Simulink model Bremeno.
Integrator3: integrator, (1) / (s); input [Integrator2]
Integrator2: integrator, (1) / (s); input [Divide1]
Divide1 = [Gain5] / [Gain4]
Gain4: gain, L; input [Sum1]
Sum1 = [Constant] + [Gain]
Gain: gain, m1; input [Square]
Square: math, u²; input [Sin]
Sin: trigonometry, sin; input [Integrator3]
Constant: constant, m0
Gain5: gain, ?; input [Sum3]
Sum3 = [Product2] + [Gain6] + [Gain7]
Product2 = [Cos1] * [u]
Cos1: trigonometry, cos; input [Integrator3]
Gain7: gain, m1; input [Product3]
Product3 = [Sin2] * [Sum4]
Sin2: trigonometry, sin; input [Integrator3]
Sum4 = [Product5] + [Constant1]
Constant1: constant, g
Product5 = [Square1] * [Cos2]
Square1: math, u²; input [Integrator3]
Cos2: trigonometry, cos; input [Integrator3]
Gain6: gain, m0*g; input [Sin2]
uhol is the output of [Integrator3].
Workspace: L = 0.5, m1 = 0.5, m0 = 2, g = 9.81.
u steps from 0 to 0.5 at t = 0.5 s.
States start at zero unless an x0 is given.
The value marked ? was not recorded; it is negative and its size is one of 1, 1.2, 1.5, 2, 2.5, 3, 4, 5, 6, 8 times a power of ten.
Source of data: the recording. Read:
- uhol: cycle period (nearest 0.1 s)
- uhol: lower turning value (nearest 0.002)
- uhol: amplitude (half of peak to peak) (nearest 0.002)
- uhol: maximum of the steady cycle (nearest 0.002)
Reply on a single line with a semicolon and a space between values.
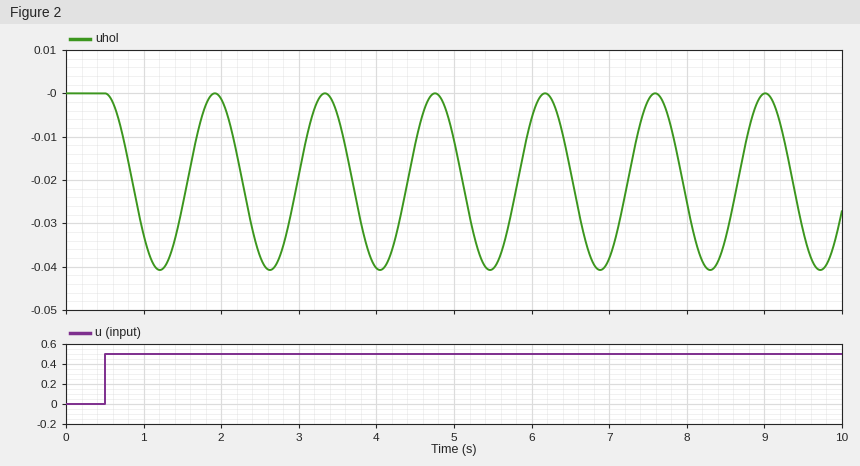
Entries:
1.4 s; -0.040; 0.020; 0.000
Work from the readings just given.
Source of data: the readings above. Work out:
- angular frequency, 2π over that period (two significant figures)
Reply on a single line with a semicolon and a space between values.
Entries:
4.5 rad/s
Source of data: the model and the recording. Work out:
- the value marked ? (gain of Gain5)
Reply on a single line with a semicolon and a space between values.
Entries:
-0.8
